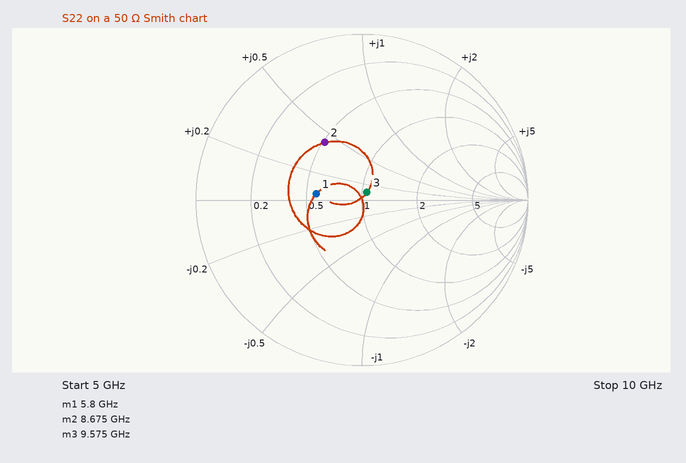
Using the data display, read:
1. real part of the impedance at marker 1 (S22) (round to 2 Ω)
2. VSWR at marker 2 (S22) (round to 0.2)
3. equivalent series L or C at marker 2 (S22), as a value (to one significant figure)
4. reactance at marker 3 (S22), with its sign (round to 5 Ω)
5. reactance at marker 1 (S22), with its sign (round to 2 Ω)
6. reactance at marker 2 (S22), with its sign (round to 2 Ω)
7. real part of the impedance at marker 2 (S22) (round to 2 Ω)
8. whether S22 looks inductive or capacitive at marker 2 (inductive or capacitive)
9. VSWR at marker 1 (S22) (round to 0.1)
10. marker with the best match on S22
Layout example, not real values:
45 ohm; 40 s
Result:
28 Ω; 2.4; 400 pH; +5 Ω; +2 Ω; +22 Ω; 26 Ω; inductive; 1.8; marker 3
